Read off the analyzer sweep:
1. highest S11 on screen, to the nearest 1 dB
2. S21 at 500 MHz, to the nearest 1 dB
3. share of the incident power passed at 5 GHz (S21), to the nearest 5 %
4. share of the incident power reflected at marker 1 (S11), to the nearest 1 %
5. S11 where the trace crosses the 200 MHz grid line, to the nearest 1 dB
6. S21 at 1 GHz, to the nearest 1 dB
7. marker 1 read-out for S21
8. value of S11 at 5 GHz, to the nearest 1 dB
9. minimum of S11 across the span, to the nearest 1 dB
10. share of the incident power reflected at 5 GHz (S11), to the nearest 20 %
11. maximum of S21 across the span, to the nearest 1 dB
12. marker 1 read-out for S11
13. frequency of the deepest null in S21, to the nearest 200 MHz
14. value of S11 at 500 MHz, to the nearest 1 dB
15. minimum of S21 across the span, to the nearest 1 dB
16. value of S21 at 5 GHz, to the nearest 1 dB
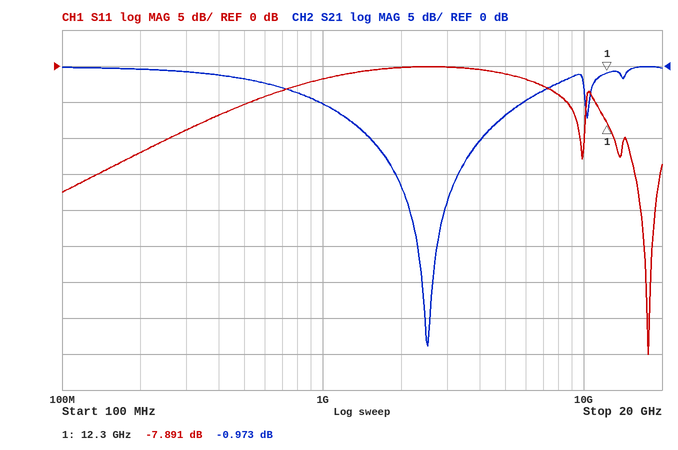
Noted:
0 dB
-2 dB
20 %
16 %
-12 dB
-5 dB
-0.973 dB
-1 dB
-40 dB
80 %
0 dB
-7.891 dB
2.6 GHz
-5 dB
-39 dB
-7 dB
